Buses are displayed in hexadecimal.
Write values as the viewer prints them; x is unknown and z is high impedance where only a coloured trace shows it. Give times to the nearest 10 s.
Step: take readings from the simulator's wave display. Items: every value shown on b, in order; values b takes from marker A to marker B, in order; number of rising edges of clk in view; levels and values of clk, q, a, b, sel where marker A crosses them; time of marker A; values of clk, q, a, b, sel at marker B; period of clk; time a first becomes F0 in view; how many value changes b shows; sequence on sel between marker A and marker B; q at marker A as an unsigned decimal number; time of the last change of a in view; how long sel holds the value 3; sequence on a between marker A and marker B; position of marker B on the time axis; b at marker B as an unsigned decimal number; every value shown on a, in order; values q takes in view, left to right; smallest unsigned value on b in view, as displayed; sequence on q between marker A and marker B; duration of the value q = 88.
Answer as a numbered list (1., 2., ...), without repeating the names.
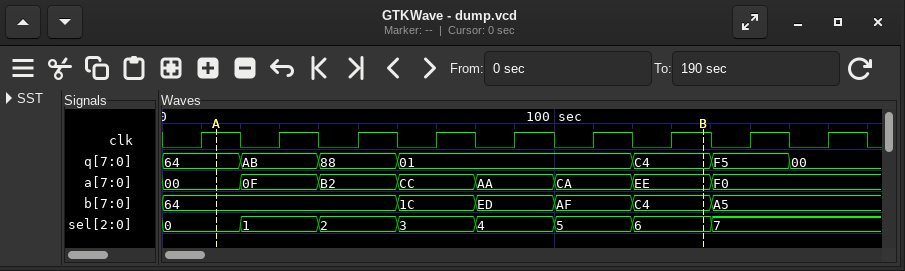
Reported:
1. 64, 1C, ED, AF, C4, A5
2. 64, 1C, ED, AF, C4
3. 9
4. clk=1, q=64, a=00, b=64, sel=0
5. 10 s
6. clk=1, q=C4, a=EE, b=C4, sel=6
7. 20 s
8. 140 s
9. 5
10. 0, 1, 2, 3, 4, 5, 6
11. 100
12. 140 s
13. 20 s
14. 00, 0F, B2, CC, AA, CA, EE
15. 140 s
16. 196
17. 00, 0F, B2, CC, AA, CA, EE, F0
18. 64, AB, 88, 01, C4, F5, 00
19. 1C
20. 64, AB, 88, 01, C4
21. 20 s
